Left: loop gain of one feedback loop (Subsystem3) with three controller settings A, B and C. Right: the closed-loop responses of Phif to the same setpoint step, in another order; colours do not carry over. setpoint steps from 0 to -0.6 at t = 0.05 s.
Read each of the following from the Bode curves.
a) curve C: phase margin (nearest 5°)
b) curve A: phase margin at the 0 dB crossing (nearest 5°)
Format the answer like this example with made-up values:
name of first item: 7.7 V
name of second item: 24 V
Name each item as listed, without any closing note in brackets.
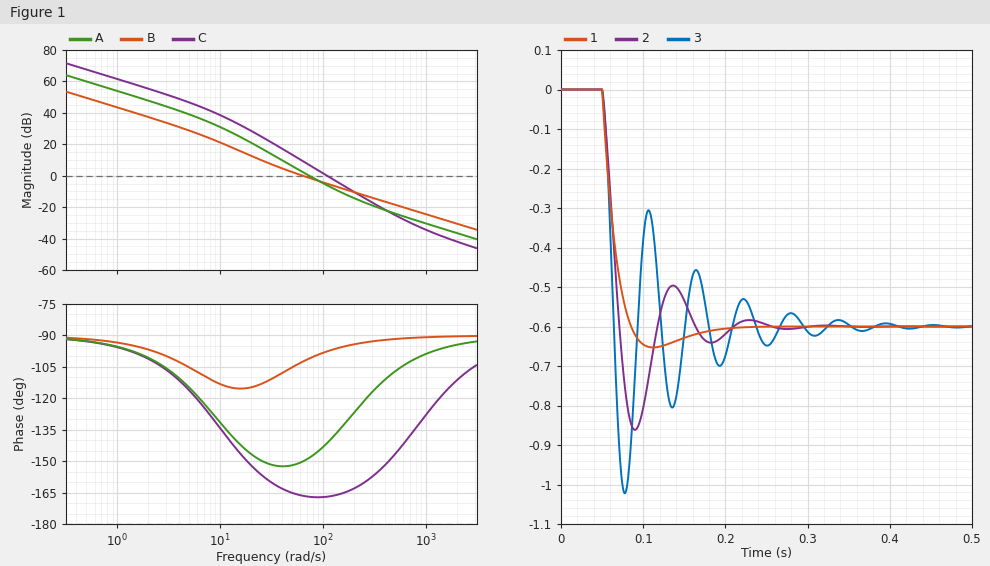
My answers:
curve C: phase margin: 15°
curve A: phase margin at the 0 dB crossing: 30°
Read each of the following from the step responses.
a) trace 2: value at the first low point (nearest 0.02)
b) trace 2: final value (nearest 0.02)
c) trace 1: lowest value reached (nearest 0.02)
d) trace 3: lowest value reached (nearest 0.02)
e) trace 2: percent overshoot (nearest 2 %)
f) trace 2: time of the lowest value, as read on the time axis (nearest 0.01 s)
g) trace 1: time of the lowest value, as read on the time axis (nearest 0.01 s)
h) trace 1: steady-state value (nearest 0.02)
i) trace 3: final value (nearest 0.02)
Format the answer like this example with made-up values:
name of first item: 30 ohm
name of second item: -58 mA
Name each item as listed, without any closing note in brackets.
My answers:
trace 2: value at the first low point: -0.86
trace 2: final value: -0.60
trace 1: lowest value reached: -0.66
trace 3: lowest value reached: -1.02
trace 2: percent overshoot: 44 %
trace 2: time of the lowest value, as read on the time axis: 0.09 s
trace 1: time of the lowest value, as read on the time axis: 0.11 s
trace 1: steady-state value: -0.60
trace 3: final value: -0.60
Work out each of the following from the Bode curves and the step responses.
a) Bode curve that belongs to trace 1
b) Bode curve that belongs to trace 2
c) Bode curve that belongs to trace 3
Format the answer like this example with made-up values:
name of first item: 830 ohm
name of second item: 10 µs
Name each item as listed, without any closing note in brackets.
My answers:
Bode curve that belongs to trace 1: B
Bode curve that belongs to trace 2: A
Bode curve that belongs to trace 3: C
